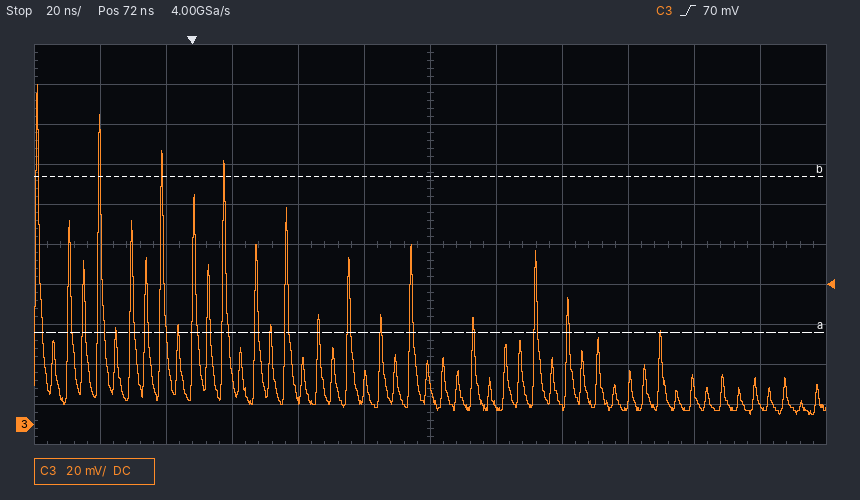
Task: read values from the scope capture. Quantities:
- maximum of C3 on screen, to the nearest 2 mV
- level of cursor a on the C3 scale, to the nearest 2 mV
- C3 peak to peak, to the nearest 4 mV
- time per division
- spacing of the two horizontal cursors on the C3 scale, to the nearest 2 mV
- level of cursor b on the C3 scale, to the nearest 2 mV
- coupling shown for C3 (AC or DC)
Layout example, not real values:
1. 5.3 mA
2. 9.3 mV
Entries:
1. 170 mV
2. 46 mV
3. 164 mV
4. 20 ns
5. 78 mV
6. 124 mV
7. DC
